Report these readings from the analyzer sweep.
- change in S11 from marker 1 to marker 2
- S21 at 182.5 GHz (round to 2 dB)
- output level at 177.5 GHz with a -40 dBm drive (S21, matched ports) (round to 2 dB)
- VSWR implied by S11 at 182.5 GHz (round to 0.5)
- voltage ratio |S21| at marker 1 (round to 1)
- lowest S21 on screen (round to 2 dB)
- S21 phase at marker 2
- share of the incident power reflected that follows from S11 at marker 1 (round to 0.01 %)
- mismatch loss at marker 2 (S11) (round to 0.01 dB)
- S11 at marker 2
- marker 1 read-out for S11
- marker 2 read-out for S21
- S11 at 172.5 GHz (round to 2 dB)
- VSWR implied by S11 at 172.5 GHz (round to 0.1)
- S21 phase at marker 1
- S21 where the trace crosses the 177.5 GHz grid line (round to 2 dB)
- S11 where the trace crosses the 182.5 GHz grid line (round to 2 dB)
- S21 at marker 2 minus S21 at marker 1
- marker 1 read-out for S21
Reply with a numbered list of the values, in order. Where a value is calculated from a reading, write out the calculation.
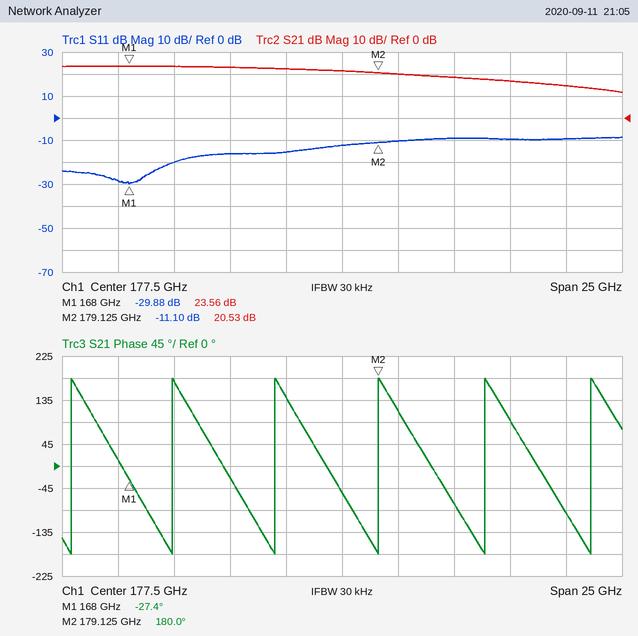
1. -11.1 − (-29.88) = 18.78 dB
2. 18 dB
3. -40 dBm + (22 dB) = -18 dBm
4. |Γ| = 10^(-10/20) = 0.3162; VSWR = (1 + 0.3162)/(1 − 0.3162) ≈ 1.92, so 2.0 to the nearest 0.5
5. 10^(23.56/20) ≈ 15
6. 12 dB
7. 180.0°
8. 10^(-29.88/10) ≈ 0.10 %
9. −10 log10(1 − 10^(-11.1/10)) ≈ 0.35 dB
10. -11.10 dB
11. -29.88 dB
12. 20.53 dB
13. -16 dB
14. |Γ| = 10^(-16/20) = 0.1585; VSWR = (1 + 0.1585)/(1 − 0.1585) ≈ 1.4
15. -27.4°
16. 22 dB
17. -10 dB
18. 20.53 − (23.56) = -3.03 dB
19. 23.56 dB
